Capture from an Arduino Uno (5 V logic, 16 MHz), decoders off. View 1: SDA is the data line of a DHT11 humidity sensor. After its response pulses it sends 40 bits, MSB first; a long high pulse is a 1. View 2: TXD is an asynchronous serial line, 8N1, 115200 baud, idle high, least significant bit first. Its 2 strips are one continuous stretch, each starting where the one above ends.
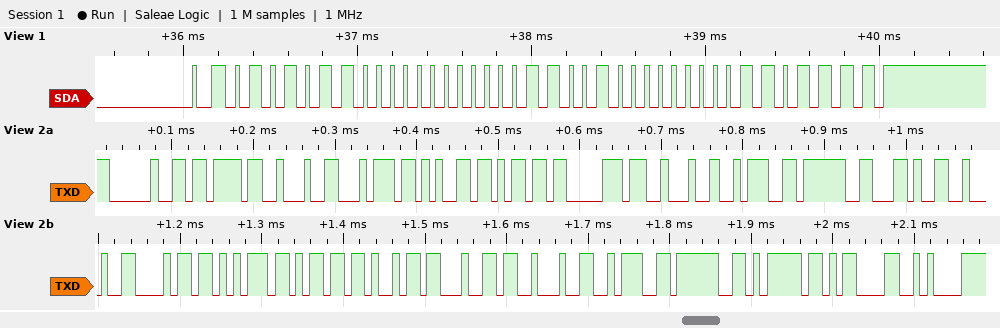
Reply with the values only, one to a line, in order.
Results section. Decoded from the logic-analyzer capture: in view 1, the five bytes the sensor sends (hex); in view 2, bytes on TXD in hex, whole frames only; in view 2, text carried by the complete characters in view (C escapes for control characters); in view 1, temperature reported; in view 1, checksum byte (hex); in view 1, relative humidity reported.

56 00 19 00 6F
20 7B 22 74 65 6D 70 22 3A 3F 2C 22 68 75 6D 69 64 22 3A 3F 7D 0D 0A
" {\"temp\":?,\"humid\":?}\r\n"
25.0 °C
0x6F
86 %
